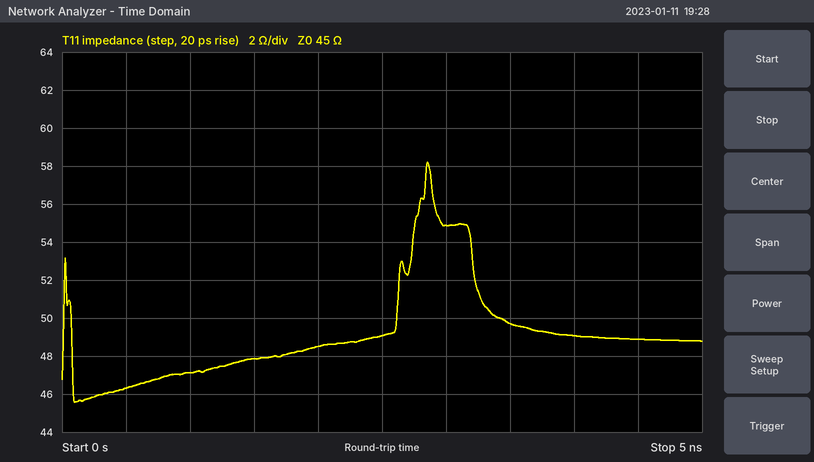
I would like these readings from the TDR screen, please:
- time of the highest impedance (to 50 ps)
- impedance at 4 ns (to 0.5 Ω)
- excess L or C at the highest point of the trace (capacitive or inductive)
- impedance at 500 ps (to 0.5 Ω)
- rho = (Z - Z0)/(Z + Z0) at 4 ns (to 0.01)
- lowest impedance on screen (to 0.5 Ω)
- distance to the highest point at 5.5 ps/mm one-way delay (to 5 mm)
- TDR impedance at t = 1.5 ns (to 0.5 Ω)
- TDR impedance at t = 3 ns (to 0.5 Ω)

2.85 ns
49.0 Ω
inductive
46.5 Ω
+0.04
45.5 Ω
260 mm
48.0 Ω
55.0 Ω
